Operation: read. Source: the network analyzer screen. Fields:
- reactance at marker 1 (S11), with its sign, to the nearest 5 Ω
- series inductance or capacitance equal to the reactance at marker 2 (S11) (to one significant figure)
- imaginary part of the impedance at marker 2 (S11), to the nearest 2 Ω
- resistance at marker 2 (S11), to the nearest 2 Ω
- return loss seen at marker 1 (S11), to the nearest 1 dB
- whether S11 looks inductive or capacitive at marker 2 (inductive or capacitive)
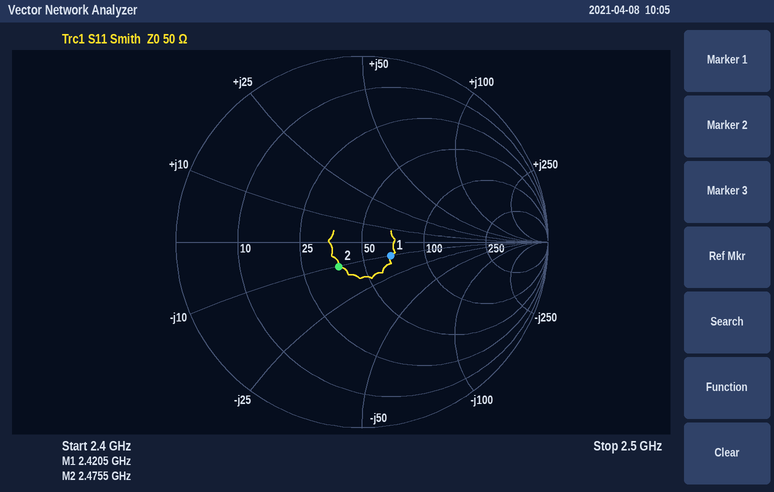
-10 Ω
6 pF
-10 Ω
38 Ω
15 dB
capacitive
